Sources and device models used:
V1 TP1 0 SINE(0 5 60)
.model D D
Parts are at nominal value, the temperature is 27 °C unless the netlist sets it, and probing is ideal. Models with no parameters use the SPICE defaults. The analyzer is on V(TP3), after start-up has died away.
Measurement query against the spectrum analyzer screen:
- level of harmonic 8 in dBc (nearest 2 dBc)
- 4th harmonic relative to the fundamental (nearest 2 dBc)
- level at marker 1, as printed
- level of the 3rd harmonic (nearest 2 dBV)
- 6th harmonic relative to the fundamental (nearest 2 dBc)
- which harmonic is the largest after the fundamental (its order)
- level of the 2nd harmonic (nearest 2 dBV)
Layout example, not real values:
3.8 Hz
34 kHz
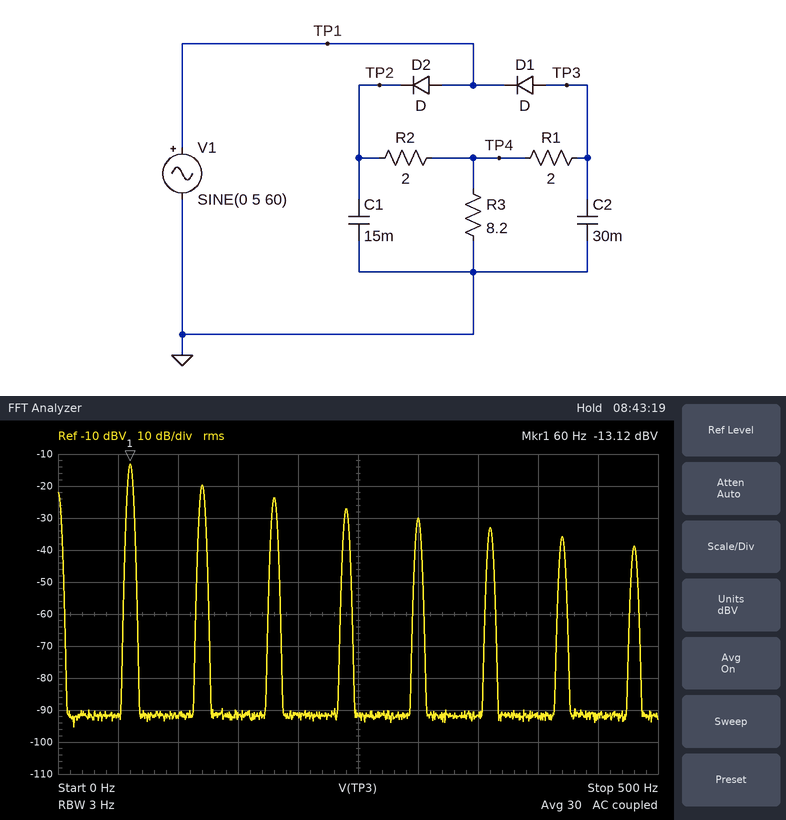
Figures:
-26 dBc
-14 dBc
-13.12 dBV
-24 dBV
-20 dBc
2
-20 dBV
